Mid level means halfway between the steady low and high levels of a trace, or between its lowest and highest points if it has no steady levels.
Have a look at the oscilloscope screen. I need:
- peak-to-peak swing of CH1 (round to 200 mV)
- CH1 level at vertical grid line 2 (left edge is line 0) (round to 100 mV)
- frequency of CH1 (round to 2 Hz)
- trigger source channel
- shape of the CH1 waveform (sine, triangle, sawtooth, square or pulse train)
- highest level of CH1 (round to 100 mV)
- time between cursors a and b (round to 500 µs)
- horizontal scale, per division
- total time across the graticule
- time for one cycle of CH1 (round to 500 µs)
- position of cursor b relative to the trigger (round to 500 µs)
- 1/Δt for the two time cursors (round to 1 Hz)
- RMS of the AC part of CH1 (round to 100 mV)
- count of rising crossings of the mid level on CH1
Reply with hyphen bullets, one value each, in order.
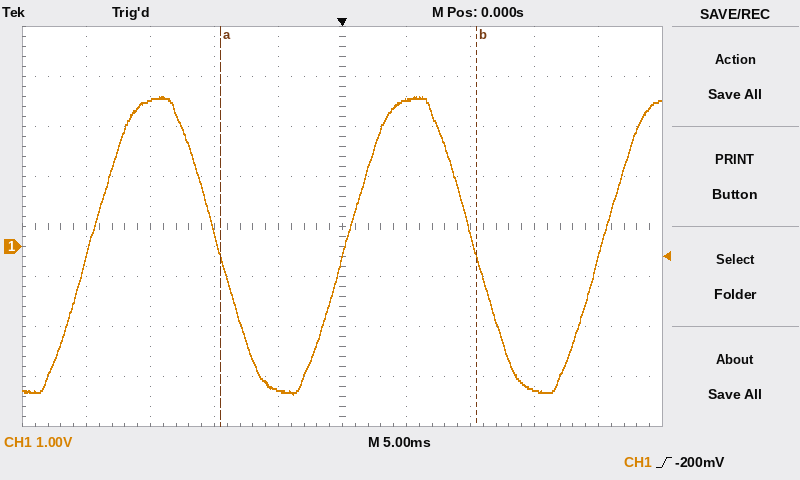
- 6.0 V
- 2.9 V
- 50 Hz
- CH1
- sine
- 3.0 V
- 20.0 ms
- 5 ms
- 50 ms
- 20.0 ms
- +10.5 ms
- 50 Hz
- 2.1 V
- 3
